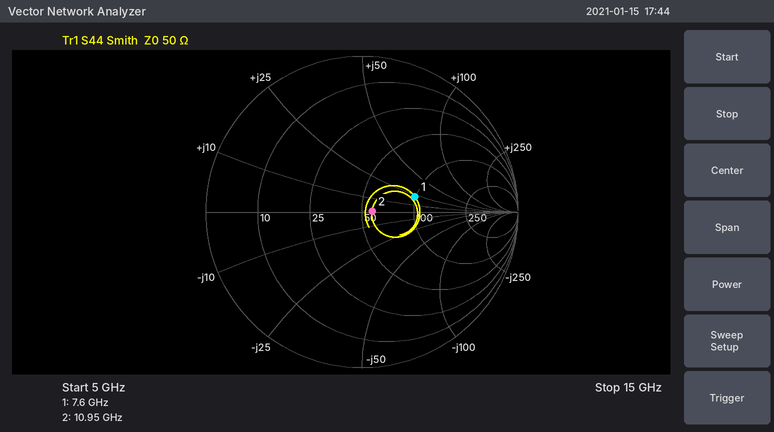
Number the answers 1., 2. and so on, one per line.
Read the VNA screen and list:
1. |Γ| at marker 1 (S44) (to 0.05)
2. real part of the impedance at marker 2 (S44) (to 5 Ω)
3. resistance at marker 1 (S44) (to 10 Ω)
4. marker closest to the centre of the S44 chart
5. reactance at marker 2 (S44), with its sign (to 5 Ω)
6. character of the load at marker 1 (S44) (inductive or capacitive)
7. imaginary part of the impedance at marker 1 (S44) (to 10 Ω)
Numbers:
1. 0.35
2. 55 Ω
3. 100 Ω
4. marker 2
5. 0 Ω
6. inductive
7. +20 Ω
